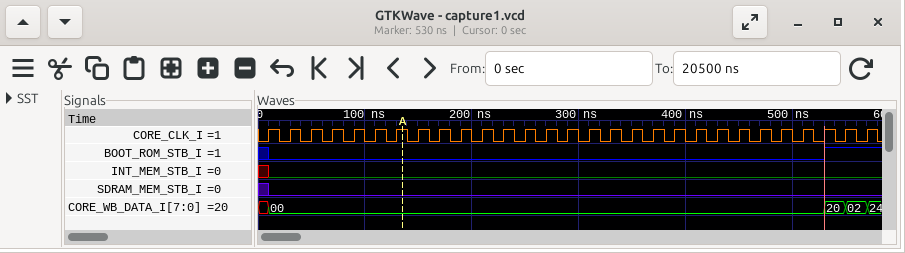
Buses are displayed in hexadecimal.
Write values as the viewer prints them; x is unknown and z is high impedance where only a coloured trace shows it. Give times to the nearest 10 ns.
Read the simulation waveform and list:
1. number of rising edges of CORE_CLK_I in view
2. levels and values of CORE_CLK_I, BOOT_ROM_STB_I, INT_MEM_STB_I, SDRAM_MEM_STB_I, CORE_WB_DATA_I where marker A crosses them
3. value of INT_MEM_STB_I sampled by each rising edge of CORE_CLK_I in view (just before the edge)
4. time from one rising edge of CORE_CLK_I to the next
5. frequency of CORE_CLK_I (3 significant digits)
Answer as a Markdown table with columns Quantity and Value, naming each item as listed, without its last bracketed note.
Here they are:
| Quantity | Value |
|---|---|
| number of rising edges of CORE_CLK_I in view | 29 |
| levels and values of CORE_CLK_I, BOOT_ROM_STB_I, INT_MEM_STB_I, SDRAM_MEM_STB_I, CORE_WB_DATA_I where marker A crosses them | CORE_CLK_I=1, BOOT_ROM_STB_I=0, INT_MEM_STB_I=0, SDRAM_MEM_STB_I=0, CORE_WB_DATA_I=00 |
| value of INT_MEM_STB_I sampled by each rising edge of CORE_CLK_I in view | x 0 0 0 0 0 0 0 0 0 0 0 0 0 0 0 0 0 0 0 0 0 0 0 0 0 0 0 0 |
| time from one rising edge of CORE_CLK_I to the next | 20 ns |
| frequency of CORE_CLK_I | 50.0 MHz |
